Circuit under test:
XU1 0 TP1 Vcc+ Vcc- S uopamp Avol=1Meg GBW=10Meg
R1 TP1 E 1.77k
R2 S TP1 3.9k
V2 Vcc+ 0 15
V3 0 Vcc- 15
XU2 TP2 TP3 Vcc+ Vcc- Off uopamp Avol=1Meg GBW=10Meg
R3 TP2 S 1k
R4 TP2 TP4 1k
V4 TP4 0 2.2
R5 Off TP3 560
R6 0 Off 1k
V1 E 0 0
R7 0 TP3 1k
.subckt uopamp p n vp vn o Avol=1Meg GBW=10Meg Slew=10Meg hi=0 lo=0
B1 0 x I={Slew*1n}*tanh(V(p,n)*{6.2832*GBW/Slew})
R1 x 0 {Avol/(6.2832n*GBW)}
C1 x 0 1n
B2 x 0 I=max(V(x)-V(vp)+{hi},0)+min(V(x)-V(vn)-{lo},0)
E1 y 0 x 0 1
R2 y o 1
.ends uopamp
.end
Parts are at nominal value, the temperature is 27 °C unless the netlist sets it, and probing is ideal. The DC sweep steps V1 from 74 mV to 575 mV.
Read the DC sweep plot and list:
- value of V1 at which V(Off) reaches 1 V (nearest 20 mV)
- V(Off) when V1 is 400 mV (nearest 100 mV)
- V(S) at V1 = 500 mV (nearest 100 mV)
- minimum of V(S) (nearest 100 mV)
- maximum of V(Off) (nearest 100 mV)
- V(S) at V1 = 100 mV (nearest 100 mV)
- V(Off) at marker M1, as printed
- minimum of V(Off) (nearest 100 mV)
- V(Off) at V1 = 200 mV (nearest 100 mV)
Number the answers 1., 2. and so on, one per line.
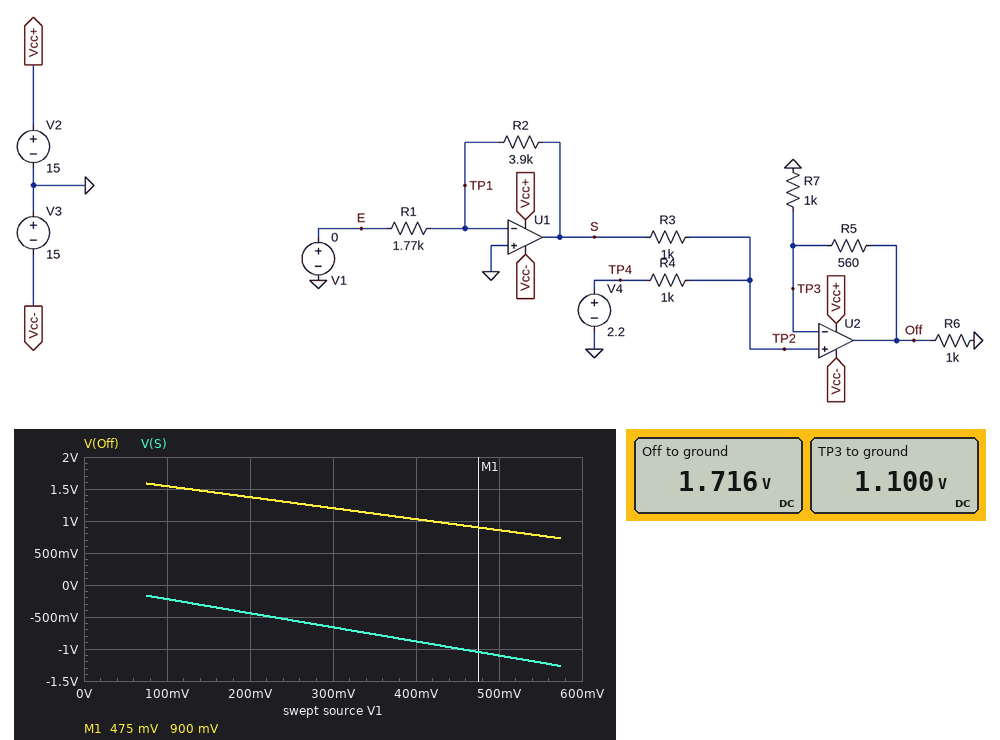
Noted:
1. 420 mV
2. 1.0 V
3. -1.1 V
4. -1.3 V
5. 1.6 V
6. -200 mV
7. 900 mV
8. 700 mV
9. 1.4 V
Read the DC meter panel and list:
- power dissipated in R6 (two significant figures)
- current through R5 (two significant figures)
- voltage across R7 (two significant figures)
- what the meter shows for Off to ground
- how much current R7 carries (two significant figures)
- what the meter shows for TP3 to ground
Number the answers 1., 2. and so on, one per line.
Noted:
1. 2.9 mW
2. 1.1 mA
3. 1.1 V
4. 1.716 V
5. 1.1 mA
6. 1.100 V
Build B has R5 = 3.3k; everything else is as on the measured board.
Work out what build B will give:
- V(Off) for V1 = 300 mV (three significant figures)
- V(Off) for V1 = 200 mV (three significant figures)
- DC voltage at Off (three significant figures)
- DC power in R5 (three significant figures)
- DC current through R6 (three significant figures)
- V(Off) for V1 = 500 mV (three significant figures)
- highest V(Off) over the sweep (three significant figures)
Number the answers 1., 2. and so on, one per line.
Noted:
1. 3.31 V
2. 3.78 V
3. 4.73 V
4. 3.99 mW
5. 4.73 mA
6. 2.36 V
7. 4.38 V
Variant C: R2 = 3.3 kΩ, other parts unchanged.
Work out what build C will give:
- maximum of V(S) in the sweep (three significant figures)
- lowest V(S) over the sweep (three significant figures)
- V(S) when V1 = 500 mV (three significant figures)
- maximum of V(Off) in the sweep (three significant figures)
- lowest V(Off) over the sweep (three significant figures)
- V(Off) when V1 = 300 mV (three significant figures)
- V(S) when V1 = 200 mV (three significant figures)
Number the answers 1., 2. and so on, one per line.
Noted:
1. -138 mV
2. -1.07 V
3. -932 mV
4. 1.61 V
5. 880 mV
6. 1.28 V
7. -373 mV
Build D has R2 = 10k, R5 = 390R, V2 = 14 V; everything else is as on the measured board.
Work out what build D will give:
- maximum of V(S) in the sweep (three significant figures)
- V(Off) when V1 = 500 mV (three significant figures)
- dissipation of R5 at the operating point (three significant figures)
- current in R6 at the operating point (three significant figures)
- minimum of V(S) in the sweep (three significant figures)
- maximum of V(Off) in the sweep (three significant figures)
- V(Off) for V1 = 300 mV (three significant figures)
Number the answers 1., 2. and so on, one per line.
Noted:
1. -418 mV
2. -434 mV
3. 472 µW
4. 1.53 mA
5. -3.25 V
6. 1.24 V
7. 351 mV
